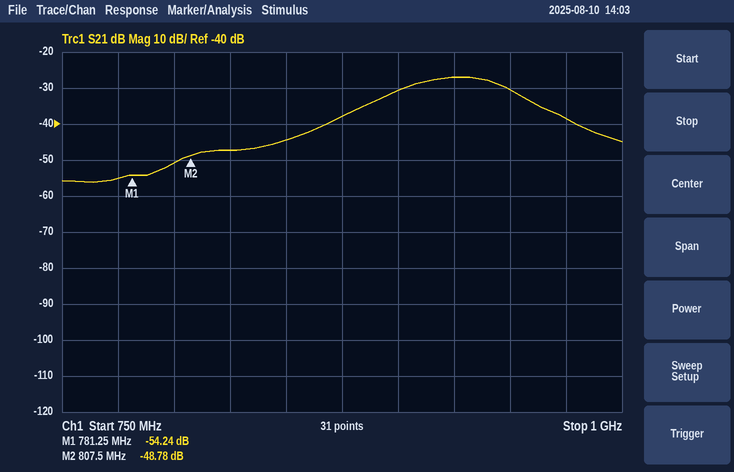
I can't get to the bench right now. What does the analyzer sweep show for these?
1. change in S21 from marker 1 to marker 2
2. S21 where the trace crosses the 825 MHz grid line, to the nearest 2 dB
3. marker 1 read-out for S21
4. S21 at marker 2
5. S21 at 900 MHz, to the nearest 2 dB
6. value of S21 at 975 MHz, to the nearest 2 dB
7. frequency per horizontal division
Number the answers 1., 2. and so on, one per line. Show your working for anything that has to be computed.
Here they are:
1. -48.78 − (-54.24) = 5.46 dB
2. -48 dB
3. -54.24 dB
4. -48.78 dB
5. -30 dB
6. -38 dB
7. 25 MHz
